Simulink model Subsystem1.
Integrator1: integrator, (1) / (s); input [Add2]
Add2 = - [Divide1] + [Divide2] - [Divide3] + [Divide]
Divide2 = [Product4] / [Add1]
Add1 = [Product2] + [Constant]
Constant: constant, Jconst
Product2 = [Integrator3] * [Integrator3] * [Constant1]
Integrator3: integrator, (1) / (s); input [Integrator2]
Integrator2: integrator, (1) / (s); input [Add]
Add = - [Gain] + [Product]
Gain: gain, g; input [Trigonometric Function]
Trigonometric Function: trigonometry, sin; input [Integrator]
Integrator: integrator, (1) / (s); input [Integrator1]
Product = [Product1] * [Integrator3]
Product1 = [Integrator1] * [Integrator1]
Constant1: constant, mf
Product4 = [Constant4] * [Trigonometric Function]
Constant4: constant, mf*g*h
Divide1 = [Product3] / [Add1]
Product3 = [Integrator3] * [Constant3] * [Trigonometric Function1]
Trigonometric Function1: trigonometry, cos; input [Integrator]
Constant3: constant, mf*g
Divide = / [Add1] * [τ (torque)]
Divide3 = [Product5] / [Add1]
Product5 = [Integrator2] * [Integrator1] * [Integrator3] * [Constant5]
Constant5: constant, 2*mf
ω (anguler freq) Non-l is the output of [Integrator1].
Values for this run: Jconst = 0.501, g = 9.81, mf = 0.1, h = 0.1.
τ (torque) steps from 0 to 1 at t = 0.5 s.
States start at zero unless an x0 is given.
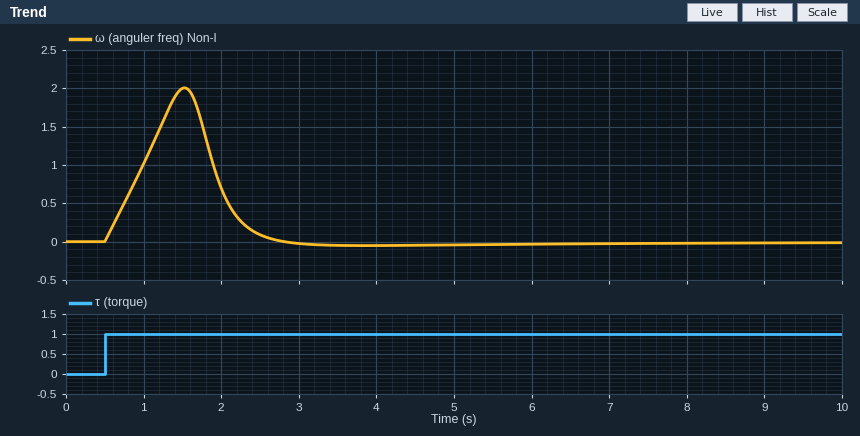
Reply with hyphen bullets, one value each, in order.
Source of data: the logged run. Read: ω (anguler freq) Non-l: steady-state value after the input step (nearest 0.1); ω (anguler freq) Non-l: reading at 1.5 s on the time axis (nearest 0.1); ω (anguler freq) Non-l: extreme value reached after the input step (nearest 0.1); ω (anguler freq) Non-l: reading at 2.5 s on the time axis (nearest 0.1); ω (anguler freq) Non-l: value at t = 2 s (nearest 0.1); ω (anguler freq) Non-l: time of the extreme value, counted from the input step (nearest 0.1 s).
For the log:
- 0.0
- 2.0
- 2.0
- 0.1
- 0.7
- 1.0 s
